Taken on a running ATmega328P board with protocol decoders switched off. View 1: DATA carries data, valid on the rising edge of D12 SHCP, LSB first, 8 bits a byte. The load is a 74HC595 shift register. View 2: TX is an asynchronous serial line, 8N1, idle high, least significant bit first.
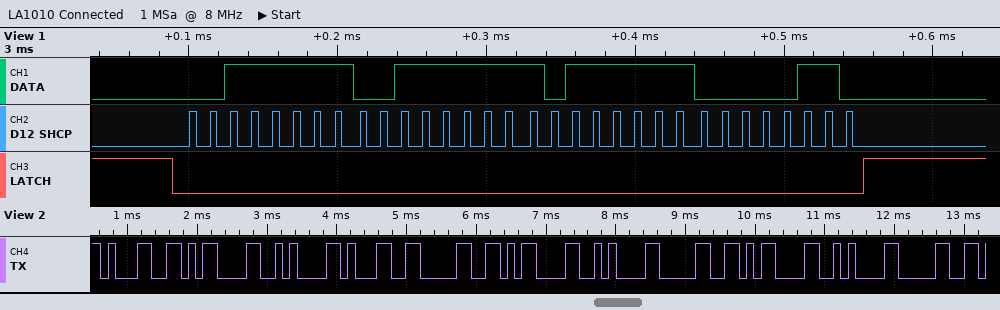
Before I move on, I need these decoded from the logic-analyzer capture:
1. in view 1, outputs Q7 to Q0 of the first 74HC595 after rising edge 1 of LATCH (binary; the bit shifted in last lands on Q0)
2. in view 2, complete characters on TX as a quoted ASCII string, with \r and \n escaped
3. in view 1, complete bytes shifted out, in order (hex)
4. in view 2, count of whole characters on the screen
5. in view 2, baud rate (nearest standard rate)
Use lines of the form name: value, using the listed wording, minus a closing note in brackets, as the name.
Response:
in view 1, outputs Q7 to Q0 of the first 74HC595 after rising edge 1 of LATCH: 00000110
in view 2, complete characters on TX as a quoted ASCII string, with \r and \n escaped: "1\r\n10\r\n0\r\n0"
in view 1, complete bytes shifted out, in order: 0xFC 0xFC 0xFD 0x60
in view 2, count of whole characters on the screen: 11
in view 2, baud rate: 9600 baud
